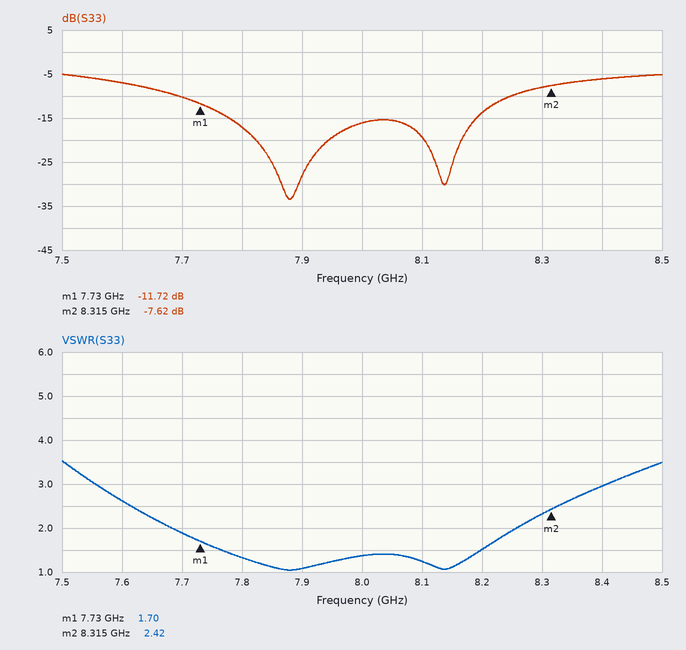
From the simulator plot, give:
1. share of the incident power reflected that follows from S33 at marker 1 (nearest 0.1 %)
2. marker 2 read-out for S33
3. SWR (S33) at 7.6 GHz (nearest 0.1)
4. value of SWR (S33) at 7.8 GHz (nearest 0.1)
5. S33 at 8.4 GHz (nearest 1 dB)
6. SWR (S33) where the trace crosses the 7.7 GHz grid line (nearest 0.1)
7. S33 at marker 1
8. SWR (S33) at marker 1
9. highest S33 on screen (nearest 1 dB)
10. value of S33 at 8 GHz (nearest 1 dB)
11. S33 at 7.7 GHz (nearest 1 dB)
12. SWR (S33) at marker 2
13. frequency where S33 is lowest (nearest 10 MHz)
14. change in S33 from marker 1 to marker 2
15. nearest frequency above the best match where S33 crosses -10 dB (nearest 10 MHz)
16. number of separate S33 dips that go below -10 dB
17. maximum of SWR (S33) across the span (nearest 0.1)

6.7 %
-7.62 dB
2.6
1.3
-6 dB
1.9
-11.72 dB
1.70
-5 dB
-16 dB
-10 dB
2.42
7.88 GHz
4.10 dB
8.25 GHz
2
3.5
